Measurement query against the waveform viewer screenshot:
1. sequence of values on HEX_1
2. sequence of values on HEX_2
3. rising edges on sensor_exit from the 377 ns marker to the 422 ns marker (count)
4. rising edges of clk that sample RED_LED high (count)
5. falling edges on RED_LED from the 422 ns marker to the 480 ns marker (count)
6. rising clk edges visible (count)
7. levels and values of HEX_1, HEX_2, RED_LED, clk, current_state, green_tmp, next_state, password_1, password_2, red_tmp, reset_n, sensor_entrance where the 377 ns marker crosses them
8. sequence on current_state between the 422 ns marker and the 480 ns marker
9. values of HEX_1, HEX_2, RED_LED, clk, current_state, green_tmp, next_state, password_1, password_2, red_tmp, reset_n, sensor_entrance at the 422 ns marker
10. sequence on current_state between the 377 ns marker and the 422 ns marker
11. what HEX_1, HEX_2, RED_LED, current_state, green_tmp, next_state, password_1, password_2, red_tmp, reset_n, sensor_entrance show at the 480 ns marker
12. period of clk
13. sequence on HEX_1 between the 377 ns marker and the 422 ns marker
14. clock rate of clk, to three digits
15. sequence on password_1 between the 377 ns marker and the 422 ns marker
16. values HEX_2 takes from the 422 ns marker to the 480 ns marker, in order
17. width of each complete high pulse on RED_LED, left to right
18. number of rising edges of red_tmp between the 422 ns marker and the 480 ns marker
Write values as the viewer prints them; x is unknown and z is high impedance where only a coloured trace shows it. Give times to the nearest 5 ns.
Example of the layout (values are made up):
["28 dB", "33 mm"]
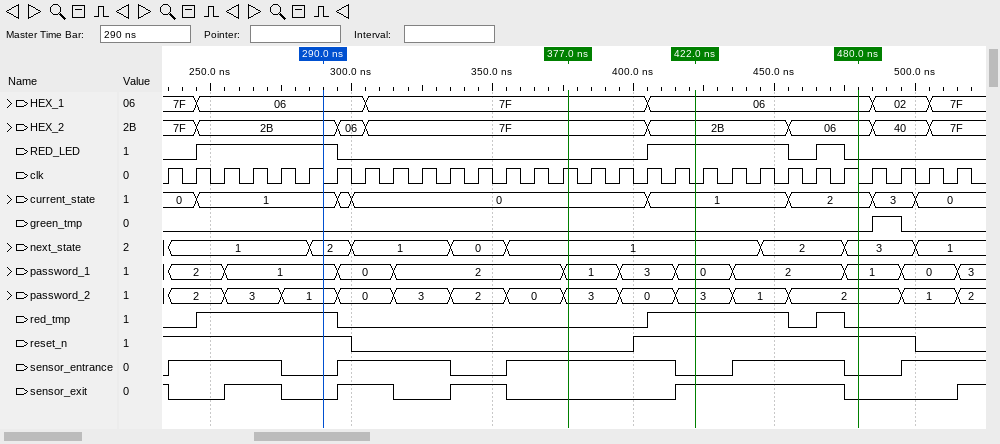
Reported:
["7F, 06, 7F, 06, 02, 7F", "7F, 2B, 06, 7F, 2B, 06, 40, 7F", "1", "11", "2", "29", "HEX_1=7F, HEX_2=7F, RED_LED=0, clk=1, current_state=0, green_tmp=0, next_state=1, password_1=1, password_2=3, red_tmp=0, reset_n=0, sensor_entrance=1", "1, 2", "HEX_1=06, HEX_2=2B, RED_LED=1, clk=0, current_state=1, green_tmp=0, next_state=1, password_1=0, password_2=3, red_tmp=1, reset_n=1, sensor_entrance=0", "0, 1", "HEX_1=06, HEX_2=06, RED_LED=0, current_state=2, green_tmp=0, next_state=3, password_1=1, password_2=2, red_tmp=0, reset_n=1, sensor_entrance=0", "10 ns", "7F, 06", "100 MHz", "1, 3, 0", "2B, 06", "50 ns, 50 ns, 10 ns", "1"]
